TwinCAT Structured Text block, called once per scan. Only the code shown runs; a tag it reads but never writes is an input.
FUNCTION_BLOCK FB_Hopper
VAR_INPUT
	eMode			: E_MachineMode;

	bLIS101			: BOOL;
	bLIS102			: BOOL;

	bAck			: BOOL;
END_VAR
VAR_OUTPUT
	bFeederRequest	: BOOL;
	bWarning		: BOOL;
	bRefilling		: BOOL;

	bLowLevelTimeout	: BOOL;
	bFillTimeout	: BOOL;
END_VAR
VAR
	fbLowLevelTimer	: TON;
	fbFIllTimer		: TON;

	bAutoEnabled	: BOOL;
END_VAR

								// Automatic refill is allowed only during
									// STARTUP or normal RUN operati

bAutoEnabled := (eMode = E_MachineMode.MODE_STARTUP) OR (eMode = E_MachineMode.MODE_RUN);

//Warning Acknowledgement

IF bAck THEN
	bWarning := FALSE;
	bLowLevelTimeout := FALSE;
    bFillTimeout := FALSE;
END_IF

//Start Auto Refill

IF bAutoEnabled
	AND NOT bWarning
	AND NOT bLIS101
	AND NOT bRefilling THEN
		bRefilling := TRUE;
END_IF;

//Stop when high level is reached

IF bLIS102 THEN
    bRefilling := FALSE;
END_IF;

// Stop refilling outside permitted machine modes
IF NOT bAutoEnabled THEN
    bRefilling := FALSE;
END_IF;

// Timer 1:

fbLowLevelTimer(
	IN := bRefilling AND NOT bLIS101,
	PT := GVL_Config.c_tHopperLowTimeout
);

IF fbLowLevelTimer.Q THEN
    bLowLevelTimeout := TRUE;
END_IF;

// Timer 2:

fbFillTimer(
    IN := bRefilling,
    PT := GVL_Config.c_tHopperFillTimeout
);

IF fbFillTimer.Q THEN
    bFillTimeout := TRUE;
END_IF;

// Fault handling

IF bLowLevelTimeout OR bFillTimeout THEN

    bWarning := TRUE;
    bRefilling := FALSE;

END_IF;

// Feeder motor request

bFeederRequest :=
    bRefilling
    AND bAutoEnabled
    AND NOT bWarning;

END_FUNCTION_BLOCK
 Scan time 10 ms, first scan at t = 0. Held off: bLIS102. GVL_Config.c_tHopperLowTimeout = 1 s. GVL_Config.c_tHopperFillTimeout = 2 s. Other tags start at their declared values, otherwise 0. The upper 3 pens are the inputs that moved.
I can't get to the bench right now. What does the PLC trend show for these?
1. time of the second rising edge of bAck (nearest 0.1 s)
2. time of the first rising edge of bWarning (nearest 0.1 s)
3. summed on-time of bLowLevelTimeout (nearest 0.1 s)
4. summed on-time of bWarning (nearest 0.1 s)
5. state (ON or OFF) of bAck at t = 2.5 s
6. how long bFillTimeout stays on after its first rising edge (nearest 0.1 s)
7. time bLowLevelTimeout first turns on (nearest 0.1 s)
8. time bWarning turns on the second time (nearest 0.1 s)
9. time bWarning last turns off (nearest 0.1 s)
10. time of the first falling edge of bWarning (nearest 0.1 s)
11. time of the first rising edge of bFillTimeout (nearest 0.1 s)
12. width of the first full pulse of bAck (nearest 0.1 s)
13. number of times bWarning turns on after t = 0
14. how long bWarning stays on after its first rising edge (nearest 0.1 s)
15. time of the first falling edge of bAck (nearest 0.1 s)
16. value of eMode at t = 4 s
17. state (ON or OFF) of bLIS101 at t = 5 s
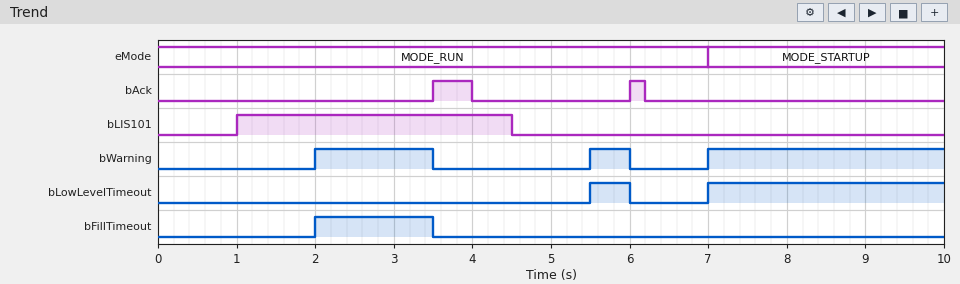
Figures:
6.0 s
2.0 s
3.5 s
5.0 s
OFF
1.5 s
5.5 s
5.5 s
6.0 s
3.5 s
2.0 s
0.5 s
3
1.5 s
4.0 s
MODE_RUN
OFF
